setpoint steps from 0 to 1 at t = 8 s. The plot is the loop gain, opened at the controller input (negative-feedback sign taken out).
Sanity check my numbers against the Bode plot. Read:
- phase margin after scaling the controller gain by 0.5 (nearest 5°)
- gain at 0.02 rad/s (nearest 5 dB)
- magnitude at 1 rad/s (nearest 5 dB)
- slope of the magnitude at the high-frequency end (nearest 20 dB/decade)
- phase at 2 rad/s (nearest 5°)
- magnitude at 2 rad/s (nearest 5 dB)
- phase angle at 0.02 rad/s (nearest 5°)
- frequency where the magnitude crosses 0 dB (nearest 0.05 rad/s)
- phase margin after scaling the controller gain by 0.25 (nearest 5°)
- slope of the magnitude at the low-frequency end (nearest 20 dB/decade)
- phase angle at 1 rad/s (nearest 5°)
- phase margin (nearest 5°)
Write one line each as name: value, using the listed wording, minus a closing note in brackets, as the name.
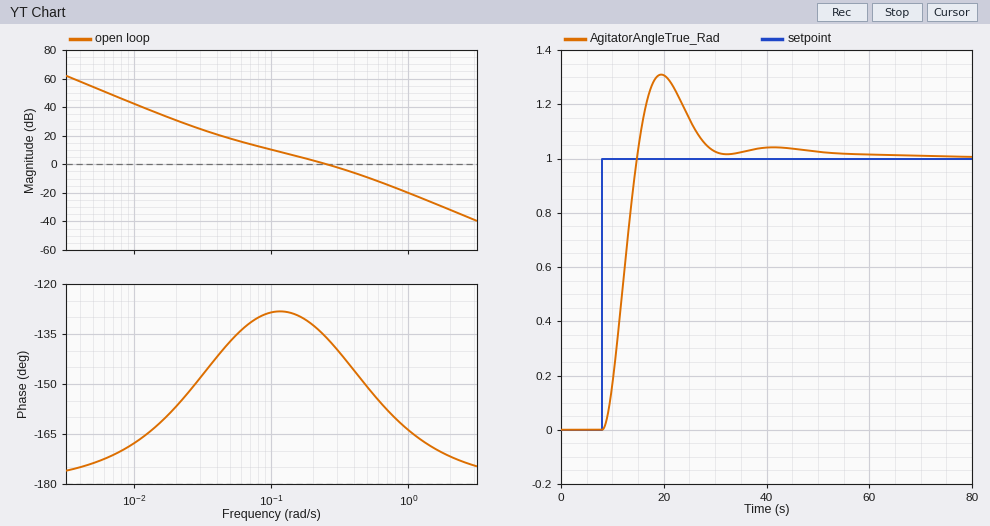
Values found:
phase margin after scaling the controller gain by 0.5: 50°
gain at 0.02 rad/s: 30 dB
magnitude at 1 rad/s: -20 dB
slope of the magnitude at the high-frequency end: -40 dB/decade
phase at 2 rad/s: -170°
magnitude at 2 rad/s: -30 dB
phase angle at 0.02 rad/s: -155°
frequency where the magnitude crosses 0 dB: 0.25 rad/s
phase margin after scaling the controller gain by 0.25: 50°
slope of the magnitude at the low-frequency end: -40 dB/decade
phase angle at 1 rad/s: -165°
phase margin: 45°
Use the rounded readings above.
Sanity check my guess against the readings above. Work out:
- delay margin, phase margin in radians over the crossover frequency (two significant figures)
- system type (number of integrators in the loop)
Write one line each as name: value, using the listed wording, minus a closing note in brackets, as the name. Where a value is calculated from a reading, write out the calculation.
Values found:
delay margin, phase margin in radians over the crossover frequency: 45 × π / 180 / 0.25 = 3.1 s
system type: 2
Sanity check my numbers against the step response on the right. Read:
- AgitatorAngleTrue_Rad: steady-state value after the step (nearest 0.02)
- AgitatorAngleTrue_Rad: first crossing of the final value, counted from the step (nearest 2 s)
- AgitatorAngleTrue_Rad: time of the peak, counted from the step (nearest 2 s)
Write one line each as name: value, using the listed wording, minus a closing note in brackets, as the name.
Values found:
AgitatorAngleTrue_Rad: steady-state value after the step: 1.00
AgitatorAngleTrue_Rad: first crossing of the final value, counted from the step: 6 s
AgitatorAngleTrue_Rad: time of the peak, counted from the step: 12 s
